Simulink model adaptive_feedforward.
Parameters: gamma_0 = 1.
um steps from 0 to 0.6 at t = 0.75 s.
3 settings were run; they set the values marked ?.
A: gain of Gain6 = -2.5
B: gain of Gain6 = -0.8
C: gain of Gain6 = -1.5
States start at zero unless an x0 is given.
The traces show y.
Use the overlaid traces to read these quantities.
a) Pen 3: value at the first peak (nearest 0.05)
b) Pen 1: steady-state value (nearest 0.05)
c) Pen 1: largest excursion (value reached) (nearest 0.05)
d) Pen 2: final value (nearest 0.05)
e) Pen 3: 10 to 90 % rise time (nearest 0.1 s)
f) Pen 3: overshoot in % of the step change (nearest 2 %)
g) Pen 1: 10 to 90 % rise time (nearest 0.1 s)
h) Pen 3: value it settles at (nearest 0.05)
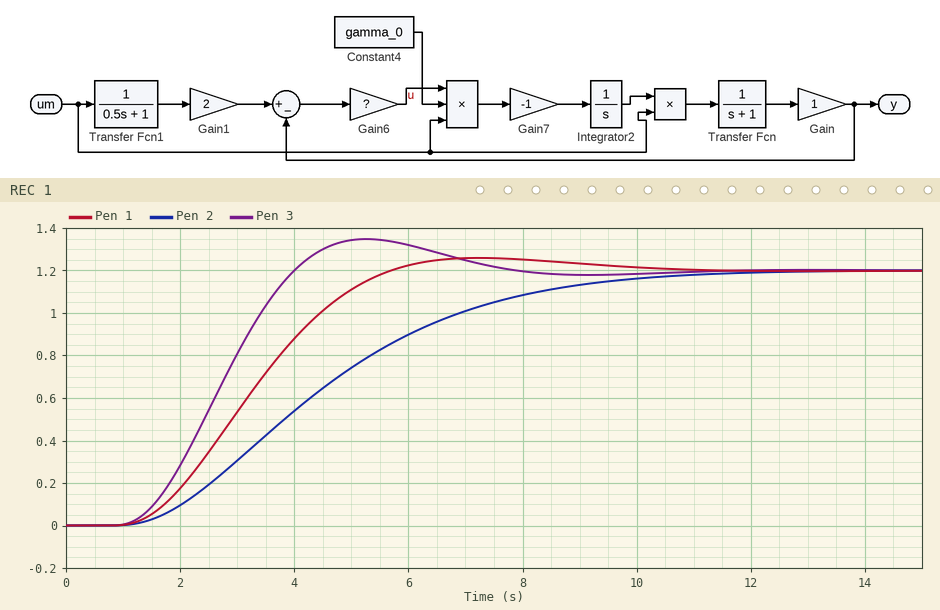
1.35
1.20
1.25
1.20
2.0 s
12 %
3.0 s
1.20
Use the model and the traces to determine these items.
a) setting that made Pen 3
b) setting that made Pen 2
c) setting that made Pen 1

A
B
C
